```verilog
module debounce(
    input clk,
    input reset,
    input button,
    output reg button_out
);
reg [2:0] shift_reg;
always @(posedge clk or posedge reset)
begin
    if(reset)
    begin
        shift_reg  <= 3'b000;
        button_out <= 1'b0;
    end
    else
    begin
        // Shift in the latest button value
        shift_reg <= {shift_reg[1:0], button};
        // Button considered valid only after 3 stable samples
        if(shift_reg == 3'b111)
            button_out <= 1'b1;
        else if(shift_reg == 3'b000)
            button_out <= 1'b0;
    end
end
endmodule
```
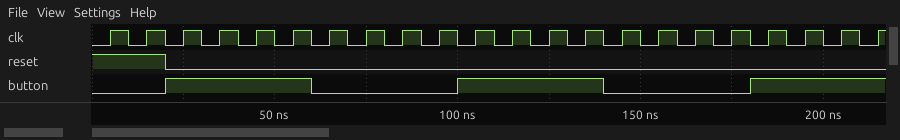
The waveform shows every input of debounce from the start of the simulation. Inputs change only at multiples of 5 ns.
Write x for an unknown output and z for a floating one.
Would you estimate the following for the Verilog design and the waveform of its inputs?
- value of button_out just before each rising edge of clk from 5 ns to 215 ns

0 0 0 0 0 0 1 1 1 1 0 0 0 0 1 1 1 1 0 0 0 0
